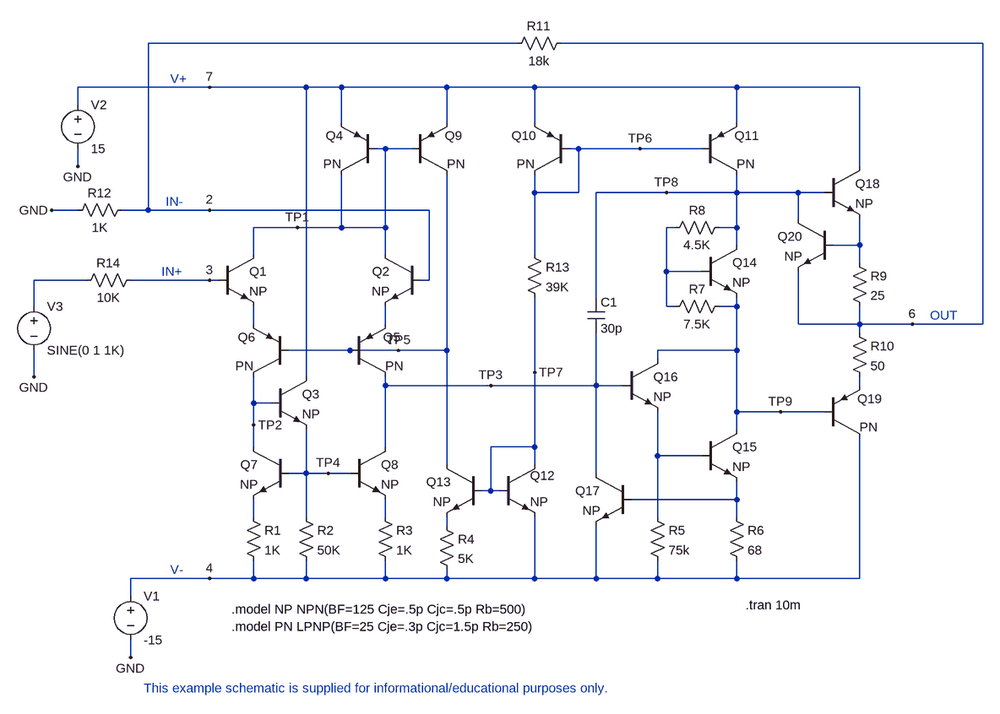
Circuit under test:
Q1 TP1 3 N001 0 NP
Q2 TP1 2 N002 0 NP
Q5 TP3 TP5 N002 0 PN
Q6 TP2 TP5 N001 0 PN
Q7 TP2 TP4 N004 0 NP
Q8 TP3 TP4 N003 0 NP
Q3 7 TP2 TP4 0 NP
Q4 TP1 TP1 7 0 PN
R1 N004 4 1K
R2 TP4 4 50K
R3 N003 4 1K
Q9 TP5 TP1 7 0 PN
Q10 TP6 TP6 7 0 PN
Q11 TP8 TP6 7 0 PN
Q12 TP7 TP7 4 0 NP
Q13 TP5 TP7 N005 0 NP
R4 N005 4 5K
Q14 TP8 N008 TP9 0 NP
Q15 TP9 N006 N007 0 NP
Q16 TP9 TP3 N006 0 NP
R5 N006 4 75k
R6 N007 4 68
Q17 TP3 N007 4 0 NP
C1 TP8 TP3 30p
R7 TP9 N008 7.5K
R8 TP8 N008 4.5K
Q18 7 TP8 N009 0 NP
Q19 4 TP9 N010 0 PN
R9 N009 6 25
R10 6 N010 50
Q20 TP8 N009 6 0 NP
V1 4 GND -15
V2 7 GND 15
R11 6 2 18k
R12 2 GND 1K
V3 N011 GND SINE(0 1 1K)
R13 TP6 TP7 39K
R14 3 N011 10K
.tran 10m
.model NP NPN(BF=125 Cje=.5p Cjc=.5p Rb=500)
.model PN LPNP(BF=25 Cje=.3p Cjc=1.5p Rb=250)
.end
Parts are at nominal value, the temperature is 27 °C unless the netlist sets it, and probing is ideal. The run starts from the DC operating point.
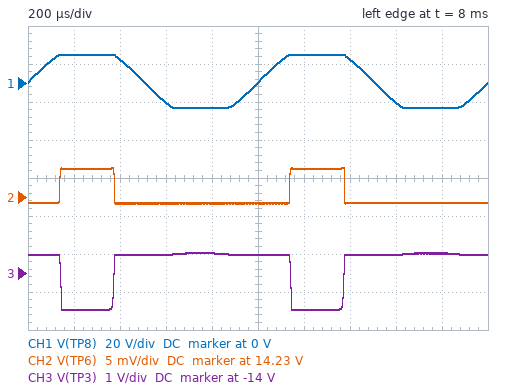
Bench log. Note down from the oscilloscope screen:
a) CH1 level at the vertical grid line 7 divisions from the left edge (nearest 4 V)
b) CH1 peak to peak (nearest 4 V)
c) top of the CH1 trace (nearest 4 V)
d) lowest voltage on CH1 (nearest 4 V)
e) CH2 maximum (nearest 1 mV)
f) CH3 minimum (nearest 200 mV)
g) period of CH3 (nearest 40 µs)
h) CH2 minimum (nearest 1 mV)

12 V
28 V
16 V
-12 V
14.234 V
-15.0 V
1.00 ms
14.229 V
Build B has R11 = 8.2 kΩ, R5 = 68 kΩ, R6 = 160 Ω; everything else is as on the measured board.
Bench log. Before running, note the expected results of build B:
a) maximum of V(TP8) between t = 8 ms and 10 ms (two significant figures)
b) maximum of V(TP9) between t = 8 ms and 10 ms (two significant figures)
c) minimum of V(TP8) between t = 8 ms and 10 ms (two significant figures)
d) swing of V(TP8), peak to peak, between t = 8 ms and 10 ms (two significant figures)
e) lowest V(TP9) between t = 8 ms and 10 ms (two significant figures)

10 V
8.8 V
-8.8 V
19 V
-10 V
